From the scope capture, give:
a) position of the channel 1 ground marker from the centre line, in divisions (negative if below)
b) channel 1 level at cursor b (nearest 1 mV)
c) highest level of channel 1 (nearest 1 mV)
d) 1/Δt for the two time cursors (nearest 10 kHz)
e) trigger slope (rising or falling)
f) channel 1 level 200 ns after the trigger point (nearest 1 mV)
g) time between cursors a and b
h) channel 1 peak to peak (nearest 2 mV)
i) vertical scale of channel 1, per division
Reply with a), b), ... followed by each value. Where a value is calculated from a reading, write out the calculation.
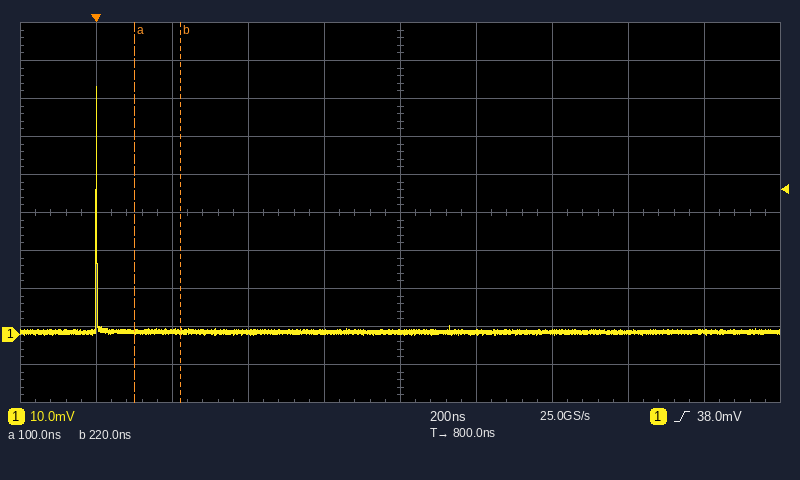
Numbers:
a) -3.2 div
b) 1 mV
c) 65 mV
d) 1 / 120 ns ≈ 8.33 MHz
e) rising
f) 1 mV
g) 220 ns − (100 ns) = 120 ns
h) 66 mV
i) 10 mV
